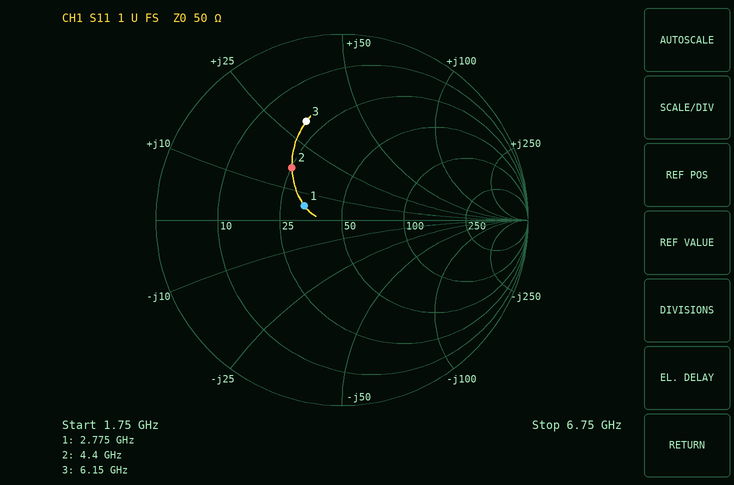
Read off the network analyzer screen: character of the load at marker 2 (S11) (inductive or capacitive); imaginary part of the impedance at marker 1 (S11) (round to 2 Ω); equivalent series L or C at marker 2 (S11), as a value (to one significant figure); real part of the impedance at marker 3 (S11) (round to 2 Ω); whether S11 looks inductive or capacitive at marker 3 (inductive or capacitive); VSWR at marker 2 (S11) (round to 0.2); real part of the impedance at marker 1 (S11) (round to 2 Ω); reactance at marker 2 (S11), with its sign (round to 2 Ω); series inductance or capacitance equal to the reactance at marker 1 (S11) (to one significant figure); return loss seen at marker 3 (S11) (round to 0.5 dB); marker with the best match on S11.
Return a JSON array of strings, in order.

["inductive", "+6 Ω", "600 pH", "20 Ω", "inductive", "2.2", "32 Ω", "+16 Ω", "300 pH", "5.0 dB", "marker 1"]
